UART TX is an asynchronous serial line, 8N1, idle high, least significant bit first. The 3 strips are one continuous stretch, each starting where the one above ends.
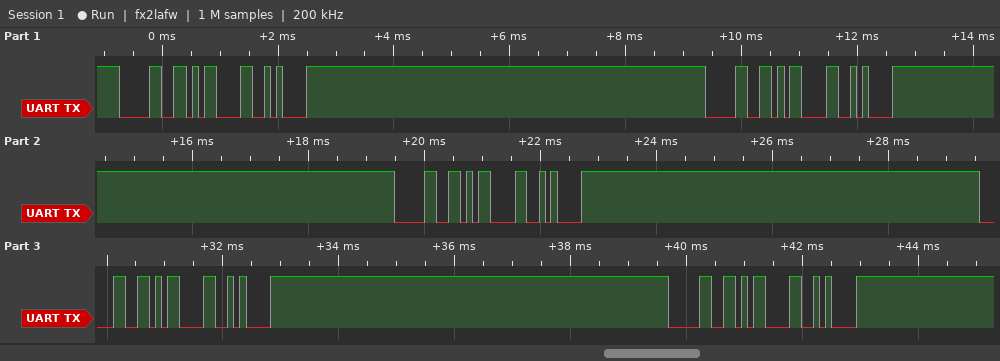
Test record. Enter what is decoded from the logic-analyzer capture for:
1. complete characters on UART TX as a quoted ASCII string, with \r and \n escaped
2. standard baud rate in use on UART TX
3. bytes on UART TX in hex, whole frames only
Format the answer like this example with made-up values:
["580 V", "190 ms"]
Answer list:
["\"0\\r\\n0\\r\\n0\\r\\n0\\r\\n0\\r\\n\"", "9600 baud", "30 0D 0A 30 0D 0A 30 0D 0A 30 0D 0A 30 0D 0A"]
